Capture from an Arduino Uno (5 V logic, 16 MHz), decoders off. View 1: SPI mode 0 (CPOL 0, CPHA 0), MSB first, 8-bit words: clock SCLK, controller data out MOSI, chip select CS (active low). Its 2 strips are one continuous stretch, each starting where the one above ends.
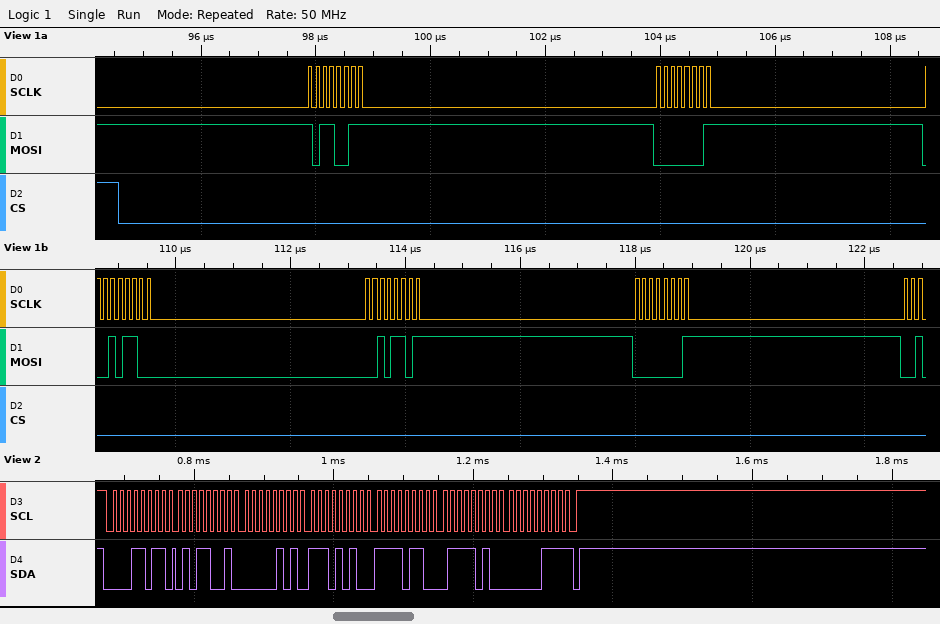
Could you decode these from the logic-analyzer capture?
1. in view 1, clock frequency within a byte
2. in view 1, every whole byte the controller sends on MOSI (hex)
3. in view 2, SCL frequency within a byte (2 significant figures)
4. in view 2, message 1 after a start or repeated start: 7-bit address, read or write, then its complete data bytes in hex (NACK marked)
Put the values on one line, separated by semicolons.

8 MHz; B3 01 2C 2D 01; 100 kHz; 0x0D read: 59 05 EA F6 7A 07 NACK
